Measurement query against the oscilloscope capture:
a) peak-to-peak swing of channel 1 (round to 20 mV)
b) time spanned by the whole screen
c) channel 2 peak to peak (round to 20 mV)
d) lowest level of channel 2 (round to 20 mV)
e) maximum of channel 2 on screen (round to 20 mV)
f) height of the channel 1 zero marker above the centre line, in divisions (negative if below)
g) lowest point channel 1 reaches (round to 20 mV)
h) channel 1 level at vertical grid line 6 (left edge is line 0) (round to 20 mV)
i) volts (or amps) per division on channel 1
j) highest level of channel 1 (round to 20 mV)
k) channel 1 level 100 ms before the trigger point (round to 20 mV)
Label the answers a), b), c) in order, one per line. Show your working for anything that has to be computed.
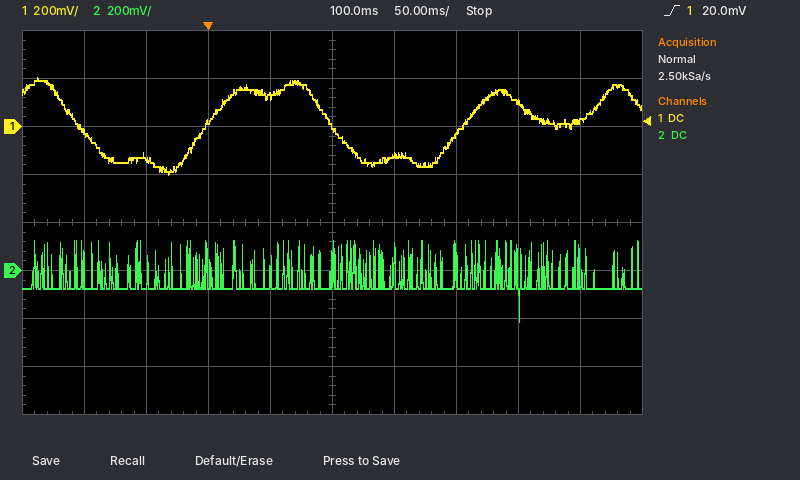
a) 200 mV − (-200 mV) = 400 mV
b) 500 ms
c) 120 mV − (-220 mV) = 340 mV
d) -220 mV
e) 120 mV
f) +2.0 div
g) -200 mV
h) -120 mV
i) 200 mV
j) 200 mV
k) -20 mV
